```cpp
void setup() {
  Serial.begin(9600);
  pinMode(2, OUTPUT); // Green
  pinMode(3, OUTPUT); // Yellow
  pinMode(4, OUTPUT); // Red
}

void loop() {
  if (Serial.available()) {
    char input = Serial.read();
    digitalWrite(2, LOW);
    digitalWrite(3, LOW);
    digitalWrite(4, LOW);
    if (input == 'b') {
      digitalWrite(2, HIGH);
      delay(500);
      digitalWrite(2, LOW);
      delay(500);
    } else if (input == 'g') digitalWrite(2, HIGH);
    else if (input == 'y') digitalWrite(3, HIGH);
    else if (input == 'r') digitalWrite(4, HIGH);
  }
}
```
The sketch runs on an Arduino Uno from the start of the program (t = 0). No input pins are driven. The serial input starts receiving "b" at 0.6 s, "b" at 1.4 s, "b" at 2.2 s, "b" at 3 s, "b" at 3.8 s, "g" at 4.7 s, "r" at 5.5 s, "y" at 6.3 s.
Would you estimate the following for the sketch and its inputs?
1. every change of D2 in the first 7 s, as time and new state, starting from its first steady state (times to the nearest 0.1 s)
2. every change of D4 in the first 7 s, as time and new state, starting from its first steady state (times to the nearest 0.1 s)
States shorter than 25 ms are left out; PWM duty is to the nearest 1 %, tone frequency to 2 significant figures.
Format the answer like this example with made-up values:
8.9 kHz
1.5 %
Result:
0 s low; 0.6 s high; 1.1 s low; 1.6 s high; 2.1 s low; 2.6 s high; 3.1 s low; 3.6 s high; 4.1 s low; 4.6 s high; 5.1 s low
0 s low; 5.6 s high; 6.3 s low
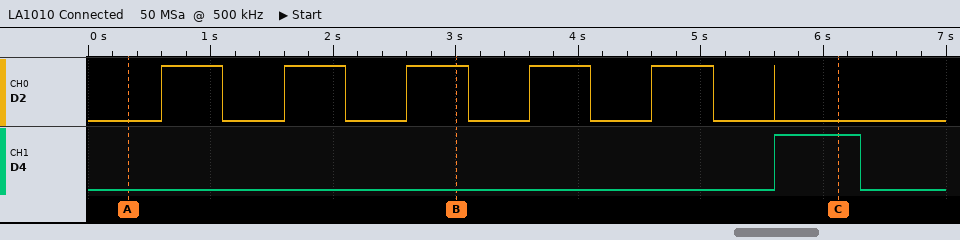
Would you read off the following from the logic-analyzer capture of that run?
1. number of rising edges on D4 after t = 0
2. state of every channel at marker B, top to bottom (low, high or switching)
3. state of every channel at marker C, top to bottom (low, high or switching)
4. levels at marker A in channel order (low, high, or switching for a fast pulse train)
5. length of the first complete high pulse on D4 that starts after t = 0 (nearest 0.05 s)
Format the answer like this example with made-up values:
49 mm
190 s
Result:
1
D2 high, D4 low
D2 low, D4 high
D2 low, D4 low
0.70 s
